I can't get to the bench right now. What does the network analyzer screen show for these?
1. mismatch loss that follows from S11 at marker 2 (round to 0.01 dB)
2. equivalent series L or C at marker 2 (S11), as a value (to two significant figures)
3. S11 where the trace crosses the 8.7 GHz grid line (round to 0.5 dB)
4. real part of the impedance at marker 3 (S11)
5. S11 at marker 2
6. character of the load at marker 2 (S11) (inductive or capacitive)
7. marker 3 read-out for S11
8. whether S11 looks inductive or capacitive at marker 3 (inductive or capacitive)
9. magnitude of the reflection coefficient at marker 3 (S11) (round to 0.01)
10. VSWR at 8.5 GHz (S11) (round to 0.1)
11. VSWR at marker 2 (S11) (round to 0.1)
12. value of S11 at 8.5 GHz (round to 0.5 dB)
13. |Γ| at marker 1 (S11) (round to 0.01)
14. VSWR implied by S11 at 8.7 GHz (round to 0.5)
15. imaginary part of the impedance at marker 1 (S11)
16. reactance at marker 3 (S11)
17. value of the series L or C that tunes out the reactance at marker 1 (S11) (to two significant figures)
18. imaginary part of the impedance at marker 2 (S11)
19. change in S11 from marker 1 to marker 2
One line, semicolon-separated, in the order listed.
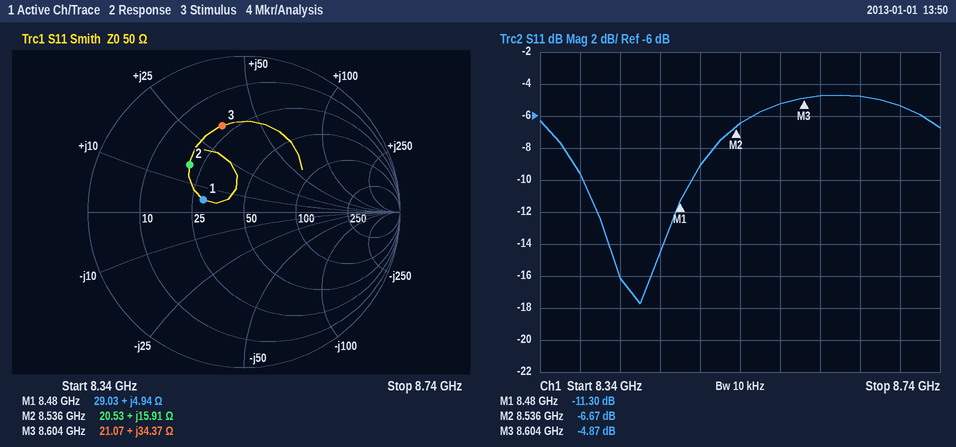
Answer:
1.05 dB; 300 pH; -5.5 dB; 21.07 Ω; -6.67 dB; inductive; -4.87 dB; inductive; 0.57; 2.1; 2.7; -9.0 dB; 0.27; 3.5; +4.94 Ω; +34.37 Ω; 3.8 pF; +15.91 Ω; 4.63 dB
